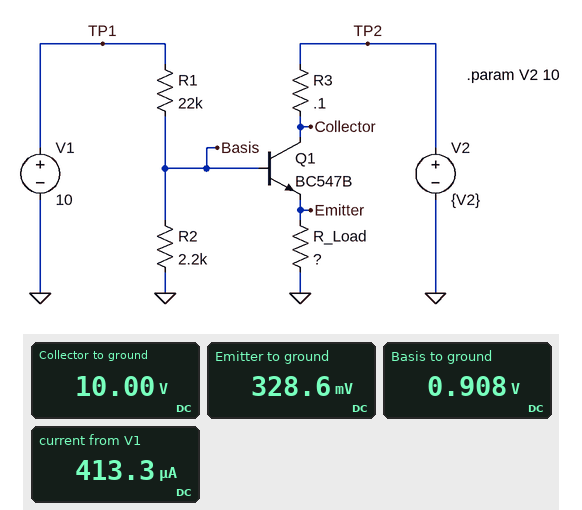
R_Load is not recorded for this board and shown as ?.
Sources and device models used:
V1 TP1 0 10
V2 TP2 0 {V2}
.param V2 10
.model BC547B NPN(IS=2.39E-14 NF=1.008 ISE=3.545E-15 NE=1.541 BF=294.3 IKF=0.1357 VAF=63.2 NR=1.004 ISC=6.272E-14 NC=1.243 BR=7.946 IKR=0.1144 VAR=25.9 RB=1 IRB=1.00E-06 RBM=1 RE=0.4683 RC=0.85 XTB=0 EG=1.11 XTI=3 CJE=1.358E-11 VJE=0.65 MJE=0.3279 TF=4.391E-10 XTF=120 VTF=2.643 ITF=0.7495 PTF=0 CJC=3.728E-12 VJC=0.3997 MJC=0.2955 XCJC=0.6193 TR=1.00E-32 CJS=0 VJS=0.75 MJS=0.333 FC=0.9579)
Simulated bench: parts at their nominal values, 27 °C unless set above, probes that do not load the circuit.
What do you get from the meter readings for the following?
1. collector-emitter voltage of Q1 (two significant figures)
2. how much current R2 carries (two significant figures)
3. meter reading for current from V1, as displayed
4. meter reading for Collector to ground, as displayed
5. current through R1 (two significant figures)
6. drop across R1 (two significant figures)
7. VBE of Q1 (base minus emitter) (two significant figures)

9.7 V
410 µA
413.3 µA
10.00 V
410 µA
9.1 V
580 mV
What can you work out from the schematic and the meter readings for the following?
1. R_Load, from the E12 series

2.7 kΩ
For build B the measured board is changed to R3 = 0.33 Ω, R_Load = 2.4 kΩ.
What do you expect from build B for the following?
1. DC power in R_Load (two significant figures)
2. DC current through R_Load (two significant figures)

44 µW
140 µA
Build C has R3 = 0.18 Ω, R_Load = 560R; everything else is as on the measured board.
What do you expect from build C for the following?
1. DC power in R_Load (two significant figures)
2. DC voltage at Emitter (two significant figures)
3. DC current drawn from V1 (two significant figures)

150 µW
290 mV
410 µA
